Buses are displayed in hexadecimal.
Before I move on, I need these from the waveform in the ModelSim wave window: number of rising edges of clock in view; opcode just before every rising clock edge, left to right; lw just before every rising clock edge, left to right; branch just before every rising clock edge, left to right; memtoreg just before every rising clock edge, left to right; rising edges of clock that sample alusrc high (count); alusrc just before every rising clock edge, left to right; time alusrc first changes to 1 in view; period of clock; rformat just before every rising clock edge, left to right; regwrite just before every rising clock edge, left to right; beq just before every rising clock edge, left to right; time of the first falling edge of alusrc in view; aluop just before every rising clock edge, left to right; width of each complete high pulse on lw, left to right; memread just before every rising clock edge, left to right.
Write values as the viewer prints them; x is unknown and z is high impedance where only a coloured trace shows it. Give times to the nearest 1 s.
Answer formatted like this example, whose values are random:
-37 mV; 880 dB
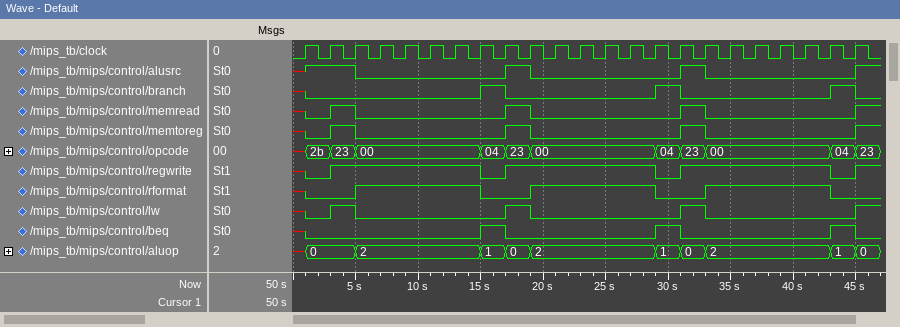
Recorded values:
23; x, 2b, 23, 00, 00, 00, 00, 00, 04, 23, 00, 00, 00, 00, 00, 04, 23, 00, 00, 00, 00, 00, 04; x 0 1 0 0 0 0 0 0 1 0 0 0 0 0 0 1 0 0 0 0 0 0; x 0 0 0 0 0 0 0 1 0 0 0 0 0 0 1 0 0 0 0 0 0 1; x 0 1 0 0 0 0 0 0 1 0 0 0 0 0 0 1 0 0 0 0 0 0; 4; x 1 1 0 0 0 0 0 0 1 0 0 0 0 0 0 1 0 0 0 0 0 0; 1 s; 2 s; x 0 0 1 1 1 1 1 0 0 1 1 1 1 1 0 0 1 1 1 1 1 0; x 0 1 1 1 1 1 1 0 1 1 1 1 1 1 0 1 1 1 1 1 1 0; x 0 0 0 0 0 0 0 1 0 0 0 0 0 0 1 0 0 0 0 0 0 1; 5 s; x, 0, 0, 2, 2, 2, 2, 2, 1, 0, 2, 2, 2, 2, 2, 1, 0, 2, 2, 2, 2, 2, 1; 2 s, 2 s, 2 s; x 0 1 0 0 0 0 0 0 1 0 0 0 0 0 0 1 0 0 0 0 0 0
